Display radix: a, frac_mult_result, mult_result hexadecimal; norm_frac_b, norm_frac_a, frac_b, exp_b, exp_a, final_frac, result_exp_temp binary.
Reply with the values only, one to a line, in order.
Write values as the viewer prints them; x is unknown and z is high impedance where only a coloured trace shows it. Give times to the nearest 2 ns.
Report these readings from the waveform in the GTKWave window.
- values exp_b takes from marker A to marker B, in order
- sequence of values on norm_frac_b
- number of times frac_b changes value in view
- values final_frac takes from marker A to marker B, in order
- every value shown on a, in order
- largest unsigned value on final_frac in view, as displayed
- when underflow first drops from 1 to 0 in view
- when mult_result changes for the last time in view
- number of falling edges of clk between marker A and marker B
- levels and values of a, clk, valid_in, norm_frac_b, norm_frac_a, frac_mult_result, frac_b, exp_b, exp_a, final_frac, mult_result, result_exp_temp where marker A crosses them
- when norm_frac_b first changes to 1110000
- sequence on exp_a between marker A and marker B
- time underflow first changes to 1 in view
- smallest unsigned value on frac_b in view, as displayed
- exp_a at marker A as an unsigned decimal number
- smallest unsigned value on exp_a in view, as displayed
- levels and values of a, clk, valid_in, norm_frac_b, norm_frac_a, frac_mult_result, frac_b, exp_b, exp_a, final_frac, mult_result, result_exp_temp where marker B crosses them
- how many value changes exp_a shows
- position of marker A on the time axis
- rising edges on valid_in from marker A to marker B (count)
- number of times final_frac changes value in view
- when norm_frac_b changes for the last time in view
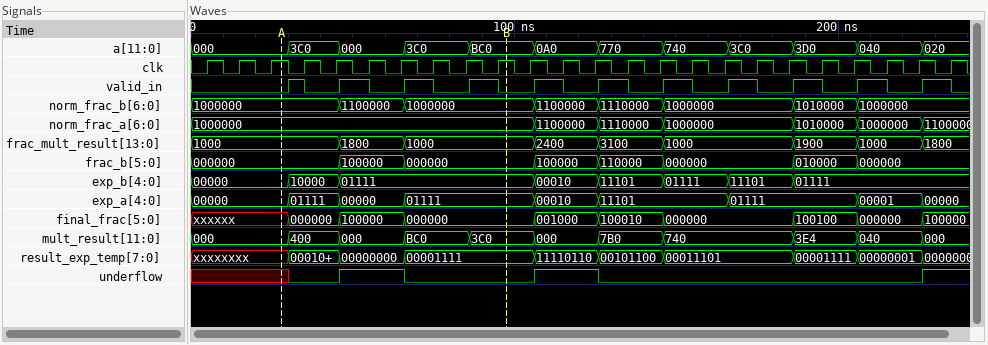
00000, 10000, 01111
1000000, 1100000, 1000000, 1100000, 1110000, 1000000, 1010000, 1000000
7
xxxxxx, 000000, 100000, 000000
000, 3C0, 000, 3C0, BC0, 0A0, 770, 740, 3C0, 3D0, 040, 020
100100
66 ns
226 ns
7
a=000, clk=1, valid_in=0, norm_frac_b=1000000, norm_frac_a=1000000, frac_mult_result=1000, frac_b=000000, exp_b=00000, exp_a=00000, final_frac=xxxxxx, mult_result=000, result_exp_temp=xxxxxxxx
126 ns
00000, 01111, 00000, 01111
46 ns
000000
0
00000
a=BC0, clk=1, valid_in=0, norm_frac_b=1000000, norm_frac_a=1000000, frac_mult_result=1000, frac_b=000000, exp_b=01111, exp_a=01111, final_frac=000000, mult_result=3C0, result_exp_temp=00001111
8
28 ns
4
9
206 ns
